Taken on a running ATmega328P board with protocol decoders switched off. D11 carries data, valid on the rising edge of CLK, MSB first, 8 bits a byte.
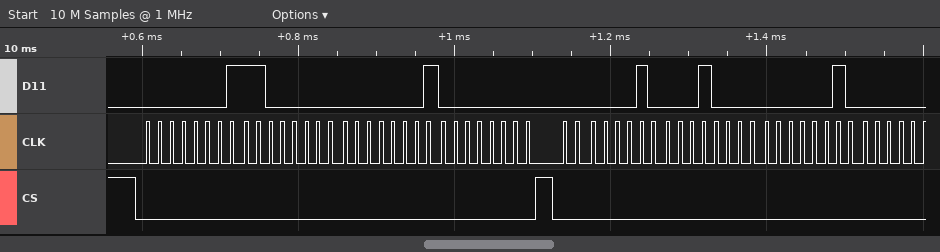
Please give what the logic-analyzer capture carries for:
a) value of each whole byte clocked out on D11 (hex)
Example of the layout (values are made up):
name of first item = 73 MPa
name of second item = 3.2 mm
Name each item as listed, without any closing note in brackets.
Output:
value of each whole byte clocked out on D11 = 0x01 0xC0 0x01 0x00 0x02 0x10 0x02
